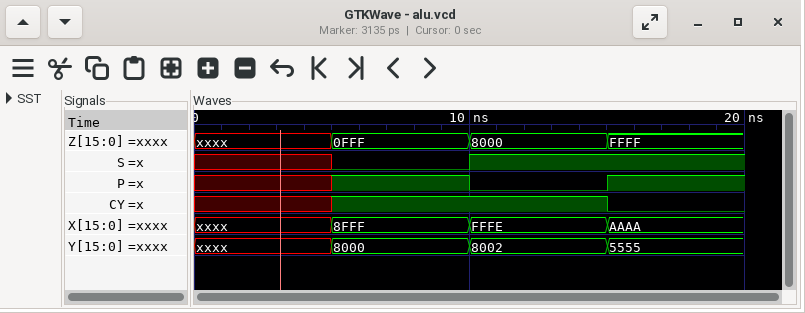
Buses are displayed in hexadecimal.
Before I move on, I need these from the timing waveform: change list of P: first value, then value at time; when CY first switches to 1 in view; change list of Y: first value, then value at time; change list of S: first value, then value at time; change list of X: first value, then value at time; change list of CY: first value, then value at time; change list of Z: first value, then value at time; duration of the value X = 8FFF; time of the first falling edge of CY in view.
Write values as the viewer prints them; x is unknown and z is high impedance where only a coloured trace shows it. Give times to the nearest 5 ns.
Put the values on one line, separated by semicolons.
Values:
x, 1 at 5 ns, 0 at 10 ns, 1 at 15 ns; 5 ns; xxxx, 8000 at 5 ns, 8002 at 10 ns, 5555 at 15 ns; x, 0 at 5 ns, 1 at 10 ns; xxxx, 8FFF at 5 ns, FFFE at 10 ns, AAAA at 15 ns; x, 1 at 5 ns, 0 at 15 ns; xxxx, 0FFF at 5 ns, 8000 at 10 ns, FFFF at 15 ns; 5 ns; 15 ns
